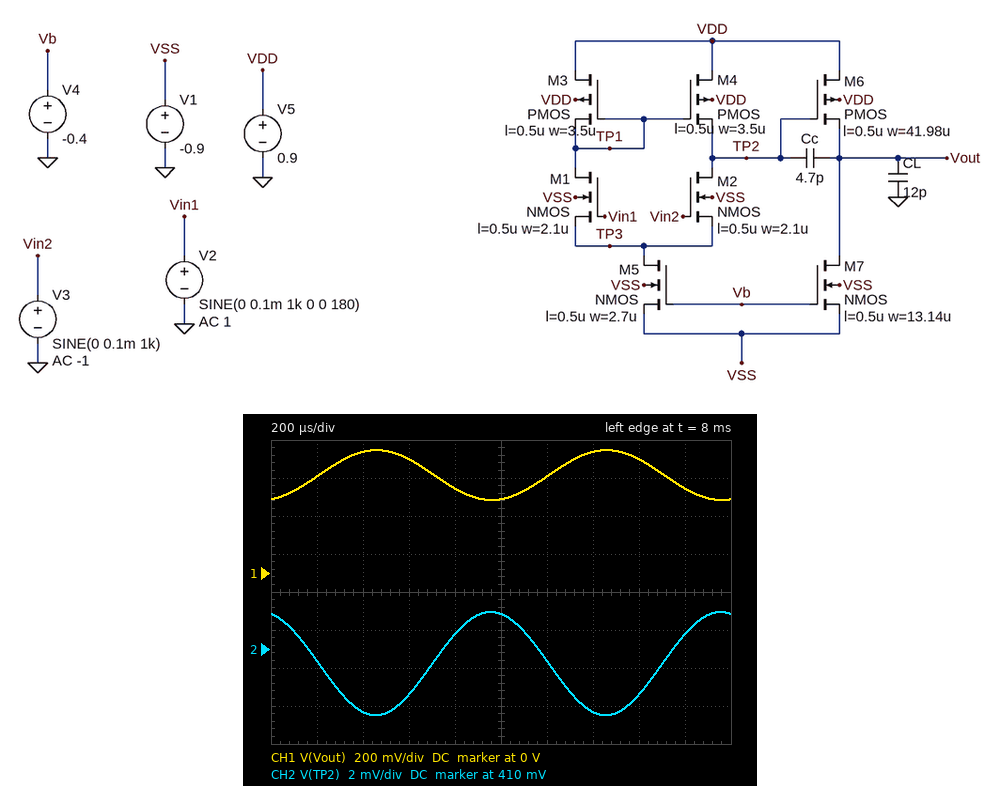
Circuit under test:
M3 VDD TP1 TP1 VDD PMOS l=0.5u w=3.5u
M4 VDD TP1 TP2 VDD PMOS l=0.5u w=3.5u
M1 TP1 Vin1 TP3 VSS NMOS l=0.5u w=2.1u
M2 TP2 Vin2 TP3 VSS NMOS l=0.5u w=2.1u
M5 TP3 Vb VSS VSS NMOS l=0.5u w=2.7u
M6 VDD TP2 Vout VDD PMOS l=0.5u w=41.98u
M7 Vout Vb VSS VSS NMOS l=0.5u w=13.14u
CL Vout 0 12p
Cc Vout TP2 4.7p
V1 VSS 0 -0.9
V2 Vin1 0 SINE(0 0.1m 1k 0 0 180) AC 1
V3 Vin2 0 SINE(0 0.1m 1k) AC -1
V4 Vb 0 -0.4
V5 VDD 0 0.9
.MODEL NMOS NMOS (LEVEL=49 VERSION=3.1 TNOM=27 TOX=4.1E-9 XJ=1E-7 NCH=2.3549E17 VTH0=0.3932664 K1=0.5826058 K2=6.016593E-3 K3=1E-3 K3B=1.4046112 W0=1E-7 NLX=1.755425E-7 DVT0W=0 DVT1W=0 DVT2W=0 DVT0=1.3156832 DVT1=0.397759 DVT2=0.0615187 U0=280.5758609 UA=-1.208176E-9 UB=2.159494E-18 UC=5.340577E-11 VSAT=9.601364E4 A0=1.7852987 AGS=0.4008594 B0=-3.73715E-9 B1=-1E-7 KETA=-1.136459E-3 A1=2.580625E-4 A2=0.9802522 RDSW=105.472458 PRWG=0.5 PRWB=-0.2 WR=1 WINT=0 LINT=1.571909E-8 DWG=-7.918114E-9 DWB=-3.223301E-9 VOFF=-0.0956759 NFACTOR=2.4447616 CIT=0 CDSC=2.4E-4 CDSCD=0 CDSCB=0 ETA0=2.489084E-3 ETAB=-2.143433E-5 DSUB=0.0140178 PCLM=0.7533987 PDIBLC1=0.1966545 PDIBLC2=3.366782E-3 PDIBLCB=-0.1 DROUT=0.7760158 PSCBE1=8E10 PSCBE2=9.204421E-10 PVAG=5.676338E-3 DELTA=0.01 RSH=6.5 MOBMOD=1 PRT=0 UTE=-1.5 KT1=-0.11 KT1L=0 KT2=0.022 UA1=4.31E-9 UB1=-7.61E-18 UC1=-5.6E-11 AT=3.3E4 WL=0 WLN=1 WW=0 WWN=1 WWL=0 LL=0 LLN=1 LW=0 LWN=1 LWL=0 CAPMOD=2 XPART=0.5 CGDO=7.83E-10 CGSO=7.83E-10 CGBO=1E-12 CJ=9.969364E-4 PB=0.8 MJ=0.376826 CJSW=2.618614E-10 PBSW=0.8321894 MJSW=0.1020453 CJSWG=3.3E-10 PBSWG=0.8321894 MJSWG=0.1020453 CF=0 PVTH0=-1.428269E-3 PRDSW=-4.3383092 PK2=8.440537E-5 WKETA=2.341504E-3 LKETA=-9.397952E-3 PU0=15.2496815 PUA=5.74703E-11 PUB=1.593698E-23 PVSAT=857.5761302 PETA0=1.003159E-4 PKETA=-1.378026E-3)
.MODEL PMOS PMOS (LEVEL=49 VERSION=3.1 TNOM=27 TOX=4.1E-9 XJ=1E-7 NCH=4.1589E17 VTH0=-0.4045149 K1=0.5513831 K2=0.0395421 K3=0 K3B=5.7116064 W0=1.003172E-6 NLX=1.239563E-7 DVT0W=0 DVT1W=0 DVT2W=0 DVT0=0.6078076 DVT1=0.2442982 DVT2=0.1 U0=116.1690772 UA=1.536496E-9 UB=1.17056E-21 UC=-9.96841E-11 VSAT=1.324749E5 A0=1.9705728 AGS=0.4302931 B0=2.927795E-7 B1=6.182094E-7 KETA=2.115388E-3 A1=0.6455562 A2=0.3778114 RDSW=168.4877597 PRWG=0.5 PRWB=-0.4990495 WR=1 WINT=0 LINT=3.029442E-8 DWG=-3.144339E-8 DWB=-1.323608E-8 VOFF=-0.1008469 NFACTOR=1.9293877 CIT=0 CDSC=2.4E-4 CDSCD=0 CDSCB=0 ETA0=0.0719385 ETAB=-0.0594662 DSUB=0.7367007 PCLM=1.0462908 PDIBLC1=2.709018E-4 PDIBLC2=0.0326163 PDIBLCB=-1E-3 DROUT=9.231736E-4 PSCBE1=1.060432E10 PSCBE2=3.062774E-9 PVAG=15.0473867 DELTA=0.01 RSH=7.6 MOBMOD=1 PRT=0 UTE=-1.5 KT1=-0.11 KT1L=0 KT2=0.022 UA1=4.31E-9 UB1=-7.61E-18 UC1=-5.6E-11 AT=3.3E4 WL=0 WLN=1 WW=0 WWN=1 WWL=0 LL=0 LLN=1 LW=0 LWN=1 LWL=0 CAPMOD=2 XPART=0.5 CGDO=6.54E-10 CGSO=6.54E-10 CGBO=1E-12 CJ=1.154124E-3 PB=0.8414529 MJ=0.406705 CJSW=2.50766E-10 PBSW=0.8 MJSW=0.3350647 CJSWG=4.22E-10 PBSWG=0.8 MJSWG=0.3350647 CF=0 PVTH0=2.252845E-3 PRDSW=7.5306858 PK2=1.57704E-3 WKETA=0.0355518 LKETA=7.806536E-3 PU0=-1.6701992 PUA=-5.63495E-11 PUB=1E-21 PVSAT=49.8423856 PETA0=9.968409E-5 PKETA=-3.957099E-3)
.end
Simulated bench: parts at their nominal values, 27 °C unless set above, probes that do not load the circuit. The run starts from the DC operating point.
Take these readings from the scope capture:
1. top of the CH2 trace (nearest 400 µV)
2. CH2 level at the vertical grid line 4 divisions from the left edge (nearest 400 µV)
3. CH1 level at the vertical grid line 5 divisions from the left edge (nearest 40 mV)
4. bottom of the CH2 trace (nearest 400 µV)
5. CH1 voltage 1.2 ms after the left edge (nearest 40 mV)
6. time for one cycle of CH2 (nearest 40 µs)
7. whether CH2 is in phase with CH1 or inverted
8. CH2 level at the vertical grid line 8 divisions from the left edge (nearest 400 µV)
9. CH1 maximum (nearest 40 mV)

412.0 mV
410.8 mV
400 mV
406.4 mV
520 mV
1.00 ms
inverted
407.6 mV
640 mV
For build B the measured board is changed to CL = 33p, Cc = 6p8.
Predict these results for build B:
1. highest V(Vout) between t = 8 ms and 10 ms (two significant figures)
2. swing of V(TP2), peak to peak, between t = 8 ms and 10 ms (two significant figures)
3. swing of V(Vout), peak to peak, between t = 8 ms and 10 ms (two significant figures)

610 mV
3.8 mV
180 mV
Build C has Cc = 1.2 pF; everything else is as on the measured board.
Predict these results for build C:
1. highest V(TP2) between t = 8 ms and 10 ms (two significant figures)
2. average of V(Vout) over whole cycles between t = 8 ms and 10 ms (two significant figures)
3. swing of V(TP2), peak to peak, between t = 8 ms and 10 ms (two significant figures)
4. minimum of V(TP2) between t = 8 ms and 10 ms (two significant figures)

420 mV
490 mV
17 mV
400 mV
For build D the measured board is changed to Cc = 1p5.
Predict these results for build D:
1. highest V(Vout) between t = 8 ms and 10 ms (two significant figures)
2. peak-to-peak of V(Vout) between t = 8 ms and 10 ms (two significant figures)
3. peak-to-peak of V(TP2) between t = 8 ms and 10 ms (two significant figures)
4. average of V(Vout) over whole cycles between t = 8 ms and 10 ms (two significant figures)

800 mV
620 mV
15 mV
500 mV
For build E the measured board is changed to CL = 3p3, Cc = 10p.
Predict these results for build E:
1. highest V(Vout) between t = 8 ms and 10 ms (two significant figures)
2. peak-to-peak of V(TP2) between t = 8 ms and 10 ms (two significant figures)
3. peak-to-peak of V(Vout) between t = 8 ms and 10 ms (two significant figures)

580 mV
2.6 mV
130 mV
